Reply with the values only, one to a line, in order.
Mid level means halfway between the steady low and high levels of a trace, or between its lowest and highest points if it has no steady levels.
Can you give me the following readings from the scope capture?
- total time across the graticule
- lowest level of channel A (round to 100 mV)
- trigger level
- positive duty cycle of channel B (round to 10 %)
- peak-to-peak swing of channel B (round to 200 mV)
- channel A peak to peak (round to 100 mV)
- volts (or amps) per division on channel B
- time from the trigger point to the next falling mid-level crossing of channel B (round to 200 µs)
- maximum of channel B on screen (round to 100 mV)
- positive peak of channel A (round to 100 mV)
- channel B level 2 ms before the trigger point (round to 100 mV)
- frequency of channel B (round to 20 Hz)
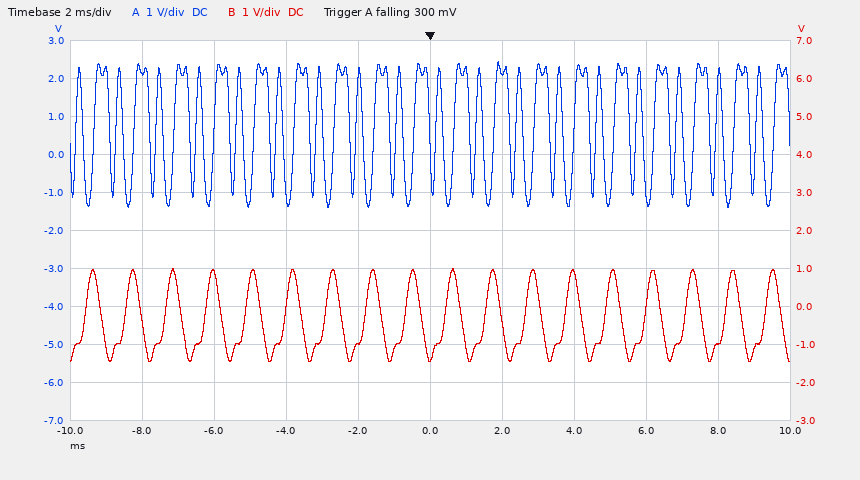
20 ms
-1.4 V
300 mV
40 %
2.4 V
3.8 V
1 V
800 µs
1.0 V
2.4 V
-1.0 V
900 Hz
